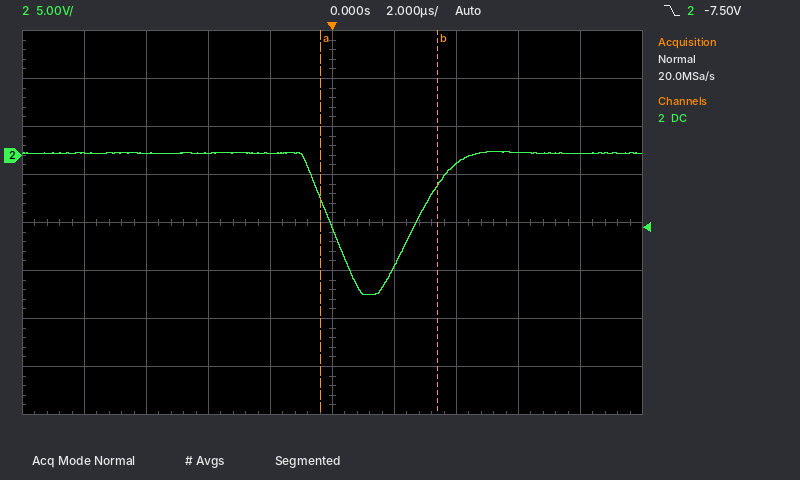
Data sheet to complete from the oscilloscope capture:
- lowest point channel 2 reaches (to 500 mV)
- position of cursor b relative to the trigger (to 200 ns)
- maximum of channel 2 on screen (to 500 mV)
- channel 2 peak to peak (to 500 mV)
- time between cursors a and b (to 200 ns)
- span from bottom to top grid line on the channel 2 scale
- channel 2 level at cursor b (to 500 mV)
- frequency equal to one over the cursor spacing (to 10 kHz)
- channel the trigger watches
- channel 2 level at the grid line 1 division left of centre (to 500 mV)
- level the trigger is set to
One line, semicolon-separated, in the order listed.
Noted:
-14.5 V; +3.4 µs; 500 mV; 15.0 V; 3.8 µs; 40 V; -3.0 V; 260 kHz; channel 2; 0.0 V; -7.50 V
